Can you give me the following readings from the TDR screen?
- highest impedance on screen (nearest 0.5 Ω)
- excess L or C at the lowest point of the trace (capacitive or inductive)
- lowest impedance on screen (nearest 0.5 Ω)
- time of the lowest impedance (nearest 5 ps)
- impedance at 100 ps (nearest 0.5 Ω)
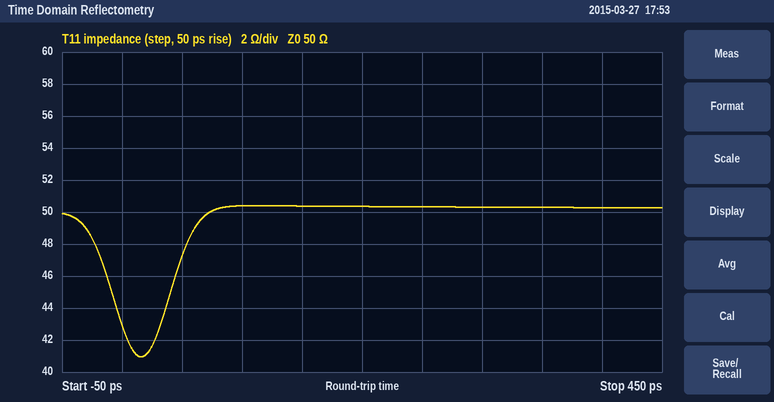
50.5 Ω
capacitive
41.0 Ω
15 ps
50.5 Ω
